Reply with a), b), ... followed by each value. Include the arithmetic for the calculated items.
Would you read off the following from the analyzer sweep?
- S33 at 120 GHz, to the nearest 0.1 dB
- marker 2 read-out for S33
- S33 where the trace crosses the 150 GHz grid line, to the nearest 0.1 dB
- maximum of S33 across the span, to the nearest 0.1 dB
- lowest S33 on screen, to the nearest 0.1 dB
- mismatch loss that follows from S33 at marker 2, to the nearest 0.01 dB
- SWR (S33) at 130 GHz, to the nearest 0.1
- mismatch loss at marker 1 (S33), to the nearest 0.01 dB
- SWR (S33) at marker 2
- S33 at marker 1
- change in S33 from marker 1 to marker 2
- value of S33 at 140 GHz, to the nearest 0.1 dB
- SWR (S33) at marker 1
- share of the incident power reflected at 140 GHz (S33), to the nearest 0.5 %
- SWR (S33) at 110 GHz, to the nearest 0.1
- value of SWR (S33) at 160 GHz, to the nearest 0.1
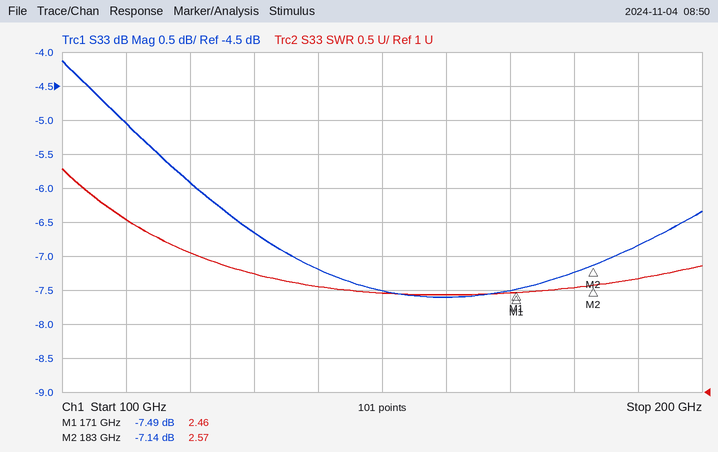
a) -5.9 dB
b) -7.14 dB
c) -7.5 dB
d) -4.1 dB
e) -7.6 dB
f) −10 log10(1 − 10^(-7.14/10)) ≈ 0.93 dB
g) 2.7
h) −10 log10(1 − 10^(-7.49/10)) ≈ 0.85 dB
i) 2.57
j) -7.49 dB
k) -7.14 − (-7.49) = 0.35 dB
l) -7.2 dB
m) 2.46
n) 10^(-7.2/10) ≈ 19.1 %, so 19.0 % to the nearest 0.5 %
o) 3.5
p) 2.4
